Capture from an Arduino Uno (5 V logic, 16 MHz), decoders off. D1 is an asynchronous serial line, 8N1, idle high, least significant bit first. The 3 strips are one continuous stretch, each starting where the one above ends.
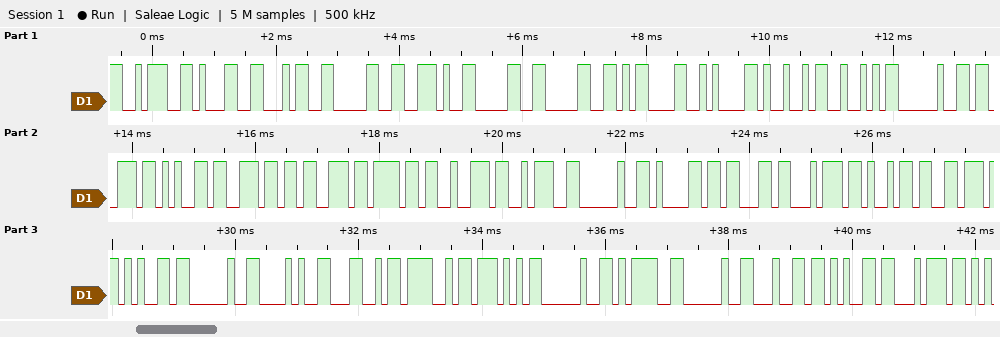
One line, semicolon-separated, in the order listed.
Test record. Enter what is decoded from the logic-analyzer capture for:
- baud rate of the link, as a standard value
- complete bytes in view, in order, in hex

9600 baud; 3A 31 34 30 2E 30 30 0D 0A 49 52 20 73 65 6E 73 6F 72 3A 20 61 63 74 69 76 65 20 28 4C 4F 57 20 3D 20 64 65 74
